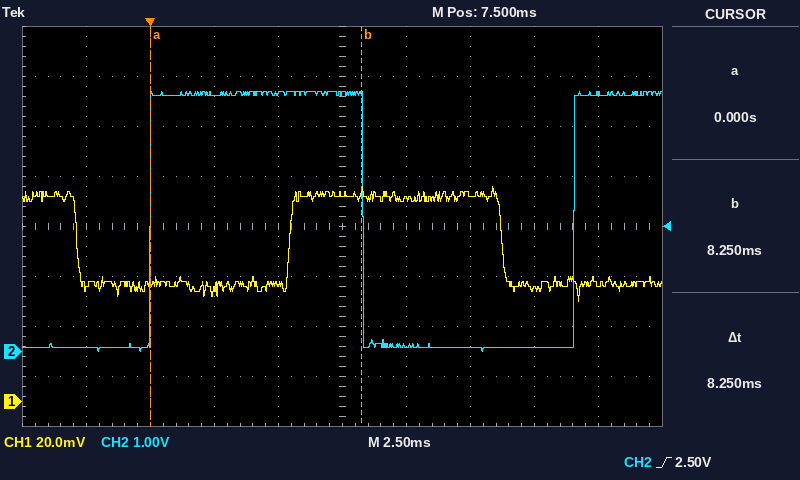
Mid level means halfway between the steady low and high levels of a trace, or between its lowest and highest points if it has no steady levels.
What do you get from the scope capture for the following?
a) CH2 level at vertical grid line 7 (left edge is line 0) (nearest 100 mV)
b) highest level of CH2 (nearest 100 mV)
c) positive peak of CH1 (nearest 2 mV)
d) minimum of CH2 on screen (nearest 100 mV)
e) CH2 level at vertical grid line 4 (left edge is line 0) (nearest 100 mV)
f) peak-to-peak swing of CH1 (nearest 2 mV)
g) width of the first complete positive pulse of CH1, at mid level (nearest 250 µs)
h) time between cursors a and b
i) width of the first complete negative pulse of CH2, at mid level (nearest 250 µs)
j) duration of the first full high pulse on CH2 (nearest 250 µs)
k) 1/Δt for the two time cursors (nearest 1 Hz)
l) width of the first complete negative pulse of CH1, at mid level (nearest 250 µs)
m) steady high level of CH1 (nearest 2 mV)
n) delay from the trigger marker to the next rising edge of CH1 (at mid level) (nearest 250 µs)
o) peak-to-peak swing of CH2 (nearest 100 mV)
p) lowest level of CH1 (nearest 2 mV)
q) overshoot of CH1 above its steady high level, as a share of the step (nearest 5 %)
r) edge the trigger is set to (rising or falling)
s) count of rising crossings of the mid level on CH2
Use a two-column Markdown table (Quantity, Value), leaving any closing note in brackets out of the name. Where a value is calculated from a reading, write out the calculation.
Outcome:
| Quantity | Value |
|---|---|
| CH2 level at vertical grid line 7 (left edge is line 0) | 100 mV |
| highest level of CH2 | 5.2 V |
| positive peak of CH1 | 86 mV |
| minimum of CH2 on screen | 0.0 V |
| CH2 level at vertical grid line 4 (left edge is line 0) | 5.2 V |
| peak-to-peak swing of CH1 | 86 mV − (40 mV) = 46 mV |
| width of the first complete positive pulse of CH1, at mid level | 8.25 ms |
| time between cursors a and b | 8.25 ms |
| width of the first complete negative pulse of CH2, at mid level | 8.25 ms |
| duration of the first full high pulse on CH2 | 8.25 ms |
| 1/Δt for the two time cursors | 1 / 8.25 ms ≈ 121 Hz |
| width of the first complete negative pulse of CH1, at mid level | 8.25 ms |
| steady high level of CH1 | 82 mV |
| delay from the trigger marker to the next rising edge of CH1 (at mid level) | 5.50 ms |
| peak-to-peak swing of CH2 | 5.2 V − (0.0 V) = 5.2 V |
| lowest level of CH1 | 40 mV |
| overshoot of CH1 above its steady high level, as a share of the step | 10 % |
| edge the trigger is set to | rising |
| count of rising crossings of the mid level on CH2 | 2 |
